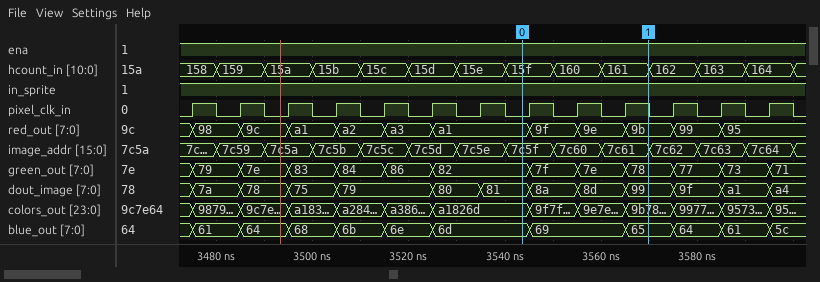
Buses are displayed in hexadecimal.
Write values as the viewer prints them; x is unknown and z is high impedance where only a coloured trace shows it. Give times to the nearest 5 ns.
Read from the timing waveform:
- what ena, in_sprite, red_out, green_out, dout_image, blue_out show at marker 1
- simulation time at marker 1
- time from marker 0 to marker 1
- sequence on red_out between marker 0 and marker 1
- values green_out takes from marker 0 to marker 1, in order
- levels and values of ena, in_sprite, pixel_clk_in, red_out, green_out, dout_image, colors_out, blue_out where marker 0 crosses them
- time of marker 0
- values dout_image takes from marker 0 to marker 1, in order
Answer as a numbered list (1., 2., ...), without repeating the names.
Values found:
1. ena=1, in_sprite=1, red_out=9b, green_out=78, dout_image=99, blue_out=65
2. 3570 ns
3. 25 ns
4. a1, 9f, 9e, 9b
5. 82, 7f, 7e, 78
6. ena=1, in_sprite=1, pixel_clk_in=0, red_out=a1, green_out=82, dout_image=81, colors_out=a1826d, blue_out=6d
7. 3545 ns
8. 81, 8a, 8d, 99
